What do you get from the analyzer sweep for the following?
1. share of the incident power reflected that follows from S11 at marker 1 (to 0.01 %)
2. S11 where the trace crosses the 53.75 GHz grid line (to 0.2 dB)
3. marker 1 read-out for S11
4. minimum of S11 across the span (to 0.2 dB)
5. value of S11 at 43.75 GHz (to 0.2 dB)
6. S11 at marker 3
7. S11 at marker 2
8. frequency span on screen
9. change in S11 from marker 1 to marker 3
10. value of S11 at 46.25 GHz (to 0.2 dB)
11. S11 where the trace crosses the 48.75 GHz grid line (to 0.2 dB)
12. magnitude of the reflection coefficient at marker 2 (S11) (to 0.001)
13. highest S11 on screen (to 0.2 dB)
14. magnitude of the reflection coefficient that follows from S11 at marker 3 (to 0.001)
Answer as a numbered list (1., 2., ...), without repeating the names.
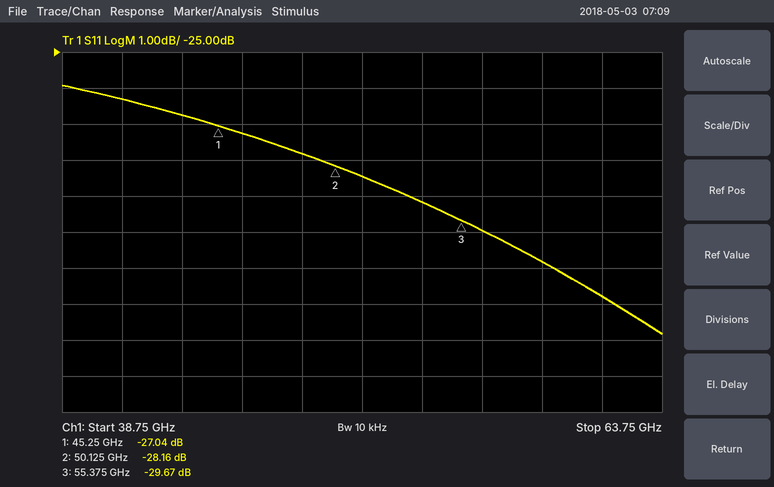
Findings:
1. 0.20 %
2. -29.2 dB
3. -27.04 dB
4. -32.8 dB
5. -26.8 dB
6. -29.67 dB
7. -28.16 dB
8. 25 GHz
9. -2.63 dB
10. -27.2 dB
11. -27.8 dB
12. 0.039
13. -26.0 dB
14. 0.033
